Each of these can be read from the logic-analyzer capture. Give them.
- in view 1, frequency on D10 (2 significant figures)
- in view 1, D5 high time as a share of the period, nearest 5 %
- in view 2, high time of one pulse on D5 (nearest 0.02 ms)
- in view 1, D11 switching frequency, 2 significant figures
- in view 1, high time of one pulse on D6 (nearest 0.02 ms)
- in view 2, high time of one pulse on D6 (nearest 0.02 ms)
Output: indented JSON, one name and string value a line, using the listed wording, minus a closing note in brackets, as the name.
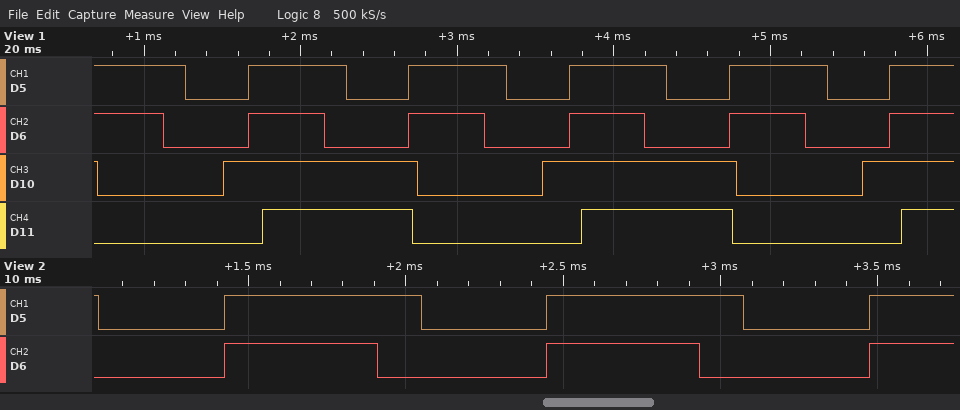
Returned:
{
  "in view 1, frequency on D10": "490 Hz",
  "in view 1, D5 high time as a share of the period, nearest 5 %": "60 %",
  "in view 2, high time of one pulse on D5": "0.62 ms",
  "in view 1, D11 switching frequency, 2 significant figures": "490 Hz",
  "in view 1, high time of one pulse on D6": "0.48 ms",
  "in view 2, high time of one pulse on D6": "0.48 ms"
}
